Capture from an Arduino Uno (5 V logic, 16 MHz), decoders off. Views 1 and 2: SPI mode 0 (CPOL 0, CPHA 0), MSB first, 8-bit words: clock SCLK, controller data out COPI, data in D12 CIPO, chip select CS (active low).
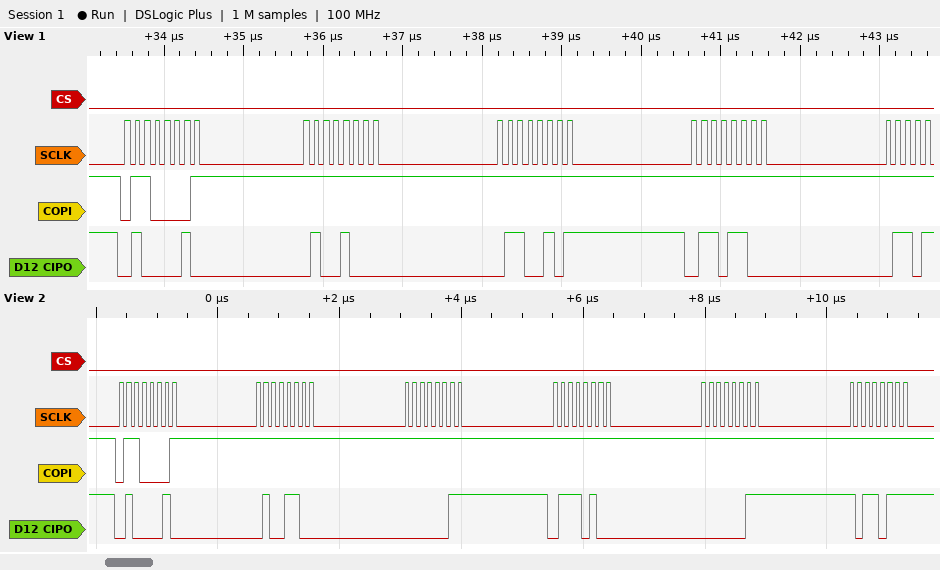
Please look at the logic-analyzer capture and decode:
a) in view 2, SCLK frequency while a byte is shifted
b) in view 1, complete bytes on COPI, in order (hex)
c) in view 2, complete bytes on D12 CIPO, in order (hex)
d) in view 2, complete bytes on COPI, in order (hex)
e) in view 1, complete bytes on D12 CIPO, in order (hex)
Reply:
8 MHz
61 FF FF FF
42 4C 03 74 03 B7
61 FF FF FF FF FF
42 48 65 6C
